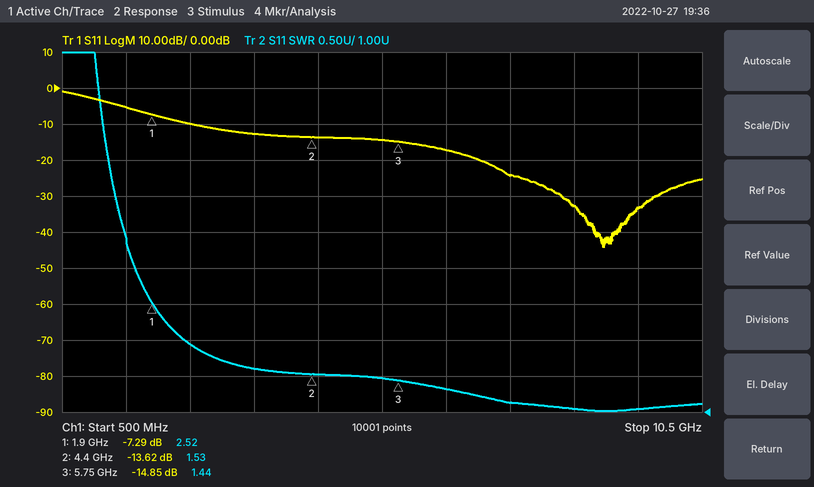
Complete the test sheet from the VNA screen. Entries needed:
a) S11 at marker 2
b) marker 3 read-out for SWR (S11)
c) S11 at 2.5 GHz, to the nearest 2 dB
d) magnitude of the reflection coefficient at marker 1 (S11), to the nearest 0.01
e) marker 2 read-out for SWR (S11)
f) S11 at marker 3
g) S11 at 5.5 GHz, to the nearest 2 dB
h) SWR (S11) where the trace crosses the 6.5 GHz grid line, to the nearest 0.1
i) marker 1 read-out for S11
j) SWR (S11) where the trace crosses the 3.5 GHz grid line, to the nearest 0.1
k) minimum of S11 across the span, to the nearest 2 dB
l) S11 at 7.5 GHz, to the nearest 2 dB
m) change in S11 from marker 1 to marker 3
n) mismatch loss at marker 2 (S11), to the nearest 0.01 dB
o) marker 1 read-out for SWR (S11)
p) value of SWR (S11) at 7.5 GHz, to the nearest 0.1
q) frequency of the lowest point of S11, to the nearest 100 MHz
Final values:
-13.62 dB
1.44
-10 dB
0.43
1.53
-14.85 dB
-14 dB
1.3
-7.29 dB
1.6
-44 dB
-24 dB
-7.56 dB
0.19 dB
2.52
1.1
9.0 GHz
